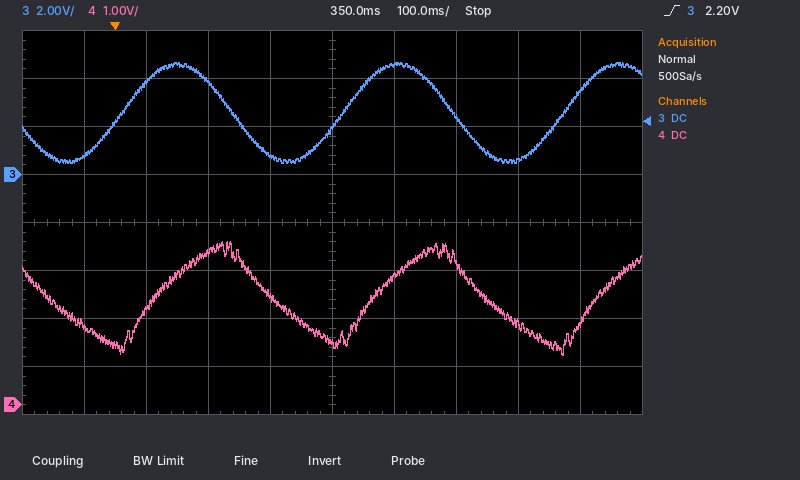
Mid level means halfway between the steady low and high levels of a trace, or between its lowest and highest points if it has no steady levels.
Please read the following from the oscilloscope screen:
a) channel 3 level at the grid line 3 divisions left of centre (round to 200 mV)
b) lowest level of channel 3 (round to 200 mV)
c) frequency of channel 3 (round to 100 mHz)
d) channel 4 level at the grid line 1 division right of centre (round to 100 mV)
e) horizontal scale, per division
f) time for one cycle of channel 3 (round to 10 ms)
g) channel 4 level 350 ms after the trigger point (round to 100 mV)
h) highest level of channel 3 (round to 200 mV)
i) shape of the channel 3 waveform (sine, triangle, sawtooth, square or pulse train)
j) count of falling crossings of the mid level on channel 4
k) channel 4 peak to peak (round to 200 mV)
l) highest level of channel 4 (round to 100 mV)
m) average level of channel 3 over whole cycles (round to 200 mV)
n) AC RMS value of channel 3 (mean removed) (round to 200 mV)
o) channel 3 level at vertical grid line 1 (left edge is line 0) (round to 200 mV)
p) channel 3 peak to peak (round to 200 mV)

3.8 V
400 mV
2.8 Hz
2.7 V
100 ms
360 ms
1.3 V
4.6 V
sine
3
2.4 V
3.4 V
2.6 V
1.4 V
800 mV
4.2 V
